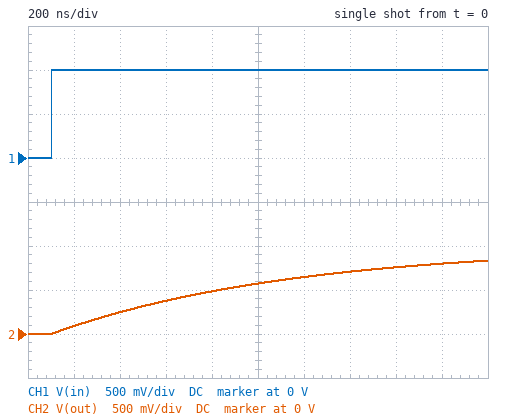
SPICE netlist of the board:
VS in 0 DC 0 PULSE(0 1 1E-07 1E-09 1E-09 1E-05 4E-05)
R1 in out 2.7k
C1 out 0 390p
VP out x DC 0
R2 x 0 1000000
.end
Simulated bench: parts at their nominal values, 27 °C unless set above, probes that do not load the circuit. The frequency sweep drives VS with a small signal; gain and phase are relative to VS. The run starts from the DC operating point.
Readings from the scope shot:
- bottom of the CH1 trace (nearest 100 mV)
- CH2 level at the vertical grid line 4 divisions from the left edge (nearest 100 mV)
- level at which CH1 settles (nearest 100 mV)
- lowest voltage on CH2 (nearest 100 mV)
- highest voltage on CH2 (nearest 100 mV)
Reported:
0 V
500 mV
1.0 V
0 V
800 mV
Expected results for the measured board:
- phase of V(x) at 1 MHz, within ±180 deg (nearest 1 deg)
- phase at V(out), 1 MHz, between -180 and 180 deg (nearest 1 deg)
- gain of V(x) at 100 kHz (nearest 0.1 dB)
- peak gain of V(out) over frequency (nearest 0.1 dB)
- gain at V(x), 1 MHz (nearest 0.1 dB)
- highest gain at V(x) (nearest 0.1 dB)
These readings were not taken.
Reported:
-81 deg
-81 deg
-1.6 dB
0 dB
-16.5 dB
0 dB
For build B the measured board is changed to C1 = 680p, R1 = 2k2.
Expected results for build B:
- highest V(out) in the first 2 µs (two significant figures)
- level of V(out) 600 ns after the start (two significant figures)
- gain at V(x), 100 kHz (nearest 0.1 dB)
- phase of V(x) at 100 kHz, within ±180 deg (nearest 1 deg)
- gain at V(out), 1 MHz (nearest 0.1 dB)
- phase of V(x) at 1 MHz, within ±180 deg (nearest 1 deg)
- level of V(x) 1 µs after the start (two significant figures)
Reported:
720 mV
280 mV
-2.8 dB
-43 deg
-19.5 dB
-84 deg
450 mV
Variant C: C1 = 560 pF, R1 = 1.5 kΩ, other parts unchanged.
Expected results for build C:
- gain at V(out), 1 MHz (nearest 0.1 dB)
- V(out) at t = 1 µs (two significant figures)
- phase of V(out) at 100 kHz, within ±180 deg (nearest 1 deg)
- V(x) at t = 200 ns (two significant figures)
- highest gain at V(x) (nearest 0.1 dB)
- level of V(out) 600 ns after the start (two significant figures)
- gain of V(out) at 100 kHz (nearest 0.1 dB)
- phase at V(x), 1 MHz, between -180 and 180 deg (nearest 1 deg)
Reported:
-14.6 dB
660 mV
-28 deg
110 mV
0 dB
450 mV
-1.1 dB
-79 deg
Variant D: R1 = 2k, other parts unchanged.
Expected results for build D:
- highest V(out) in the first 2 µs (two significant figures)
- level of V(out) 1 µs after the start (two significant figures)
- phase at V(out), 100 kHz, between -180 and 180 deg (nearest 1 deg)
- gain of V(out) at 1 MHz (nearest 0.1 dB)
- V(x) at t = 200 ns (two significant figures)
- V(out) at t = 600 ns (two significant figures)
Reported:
910 mV
680 mV
-26 deg
-14.0 dB
120 mV
470 mV
